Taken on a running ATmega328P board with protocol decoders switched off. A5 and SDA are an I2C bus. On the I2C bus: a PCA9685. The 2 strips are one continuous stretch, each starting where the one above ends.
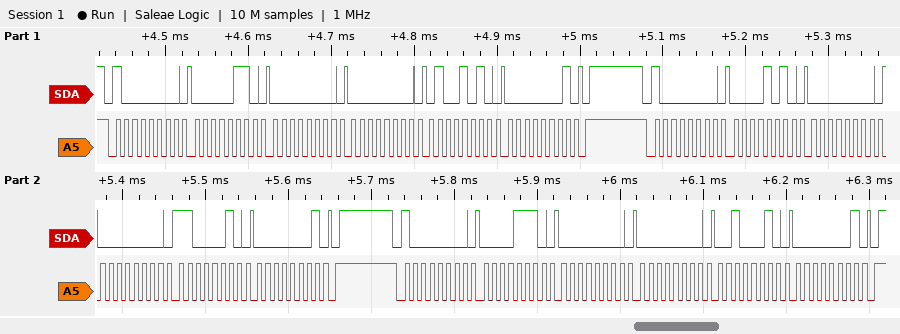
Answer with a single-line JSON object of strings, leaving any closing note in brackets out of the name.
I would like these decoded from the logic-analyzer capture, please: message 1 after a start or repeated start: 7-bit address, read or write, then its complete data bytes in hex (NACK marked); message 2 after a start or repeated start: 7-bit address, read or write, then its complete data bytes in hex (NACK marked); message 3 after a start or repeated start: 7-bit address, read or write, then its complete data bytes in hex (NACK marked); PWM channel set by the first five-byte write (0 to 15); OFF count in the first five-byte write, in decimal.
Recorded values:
{"message 1 after a start or repeated start: 7-bit address, read or write, then its complete data bytes in hex": "0x40 write: 06 00 00 4A 01", "message 2 after a start or repeated start: 7-bit address, read or write, then its complete data bytes in hex": "0x40 write: 0A 00 00 C2 01", "message 3 after a start or repeated start: 7-bit address, read or write, then its complete data bytes in hex": "0x40 write: 0E 00 00 22 01", "PWM channel set by the first five-byte write": "0", "OFF count in the first five-byte write, in decimal": "330"}
